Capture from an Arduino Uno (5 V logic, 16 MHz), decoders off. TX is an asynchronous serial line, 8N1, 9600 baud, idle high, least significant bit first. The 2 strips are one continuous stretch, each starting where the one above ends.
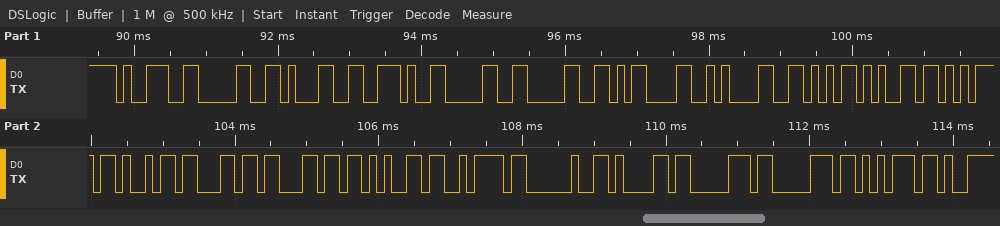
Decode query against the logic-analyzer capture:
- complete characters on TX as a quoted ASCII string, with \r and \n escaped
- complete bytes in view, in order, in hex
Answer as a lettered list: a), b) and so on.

a) "901.00\r\nVeuillez appu"
b) 39 30 31 2E 30 30 0D 0A 56 65 75 69 6C 6C 65 7A 20 61 70 70 75
